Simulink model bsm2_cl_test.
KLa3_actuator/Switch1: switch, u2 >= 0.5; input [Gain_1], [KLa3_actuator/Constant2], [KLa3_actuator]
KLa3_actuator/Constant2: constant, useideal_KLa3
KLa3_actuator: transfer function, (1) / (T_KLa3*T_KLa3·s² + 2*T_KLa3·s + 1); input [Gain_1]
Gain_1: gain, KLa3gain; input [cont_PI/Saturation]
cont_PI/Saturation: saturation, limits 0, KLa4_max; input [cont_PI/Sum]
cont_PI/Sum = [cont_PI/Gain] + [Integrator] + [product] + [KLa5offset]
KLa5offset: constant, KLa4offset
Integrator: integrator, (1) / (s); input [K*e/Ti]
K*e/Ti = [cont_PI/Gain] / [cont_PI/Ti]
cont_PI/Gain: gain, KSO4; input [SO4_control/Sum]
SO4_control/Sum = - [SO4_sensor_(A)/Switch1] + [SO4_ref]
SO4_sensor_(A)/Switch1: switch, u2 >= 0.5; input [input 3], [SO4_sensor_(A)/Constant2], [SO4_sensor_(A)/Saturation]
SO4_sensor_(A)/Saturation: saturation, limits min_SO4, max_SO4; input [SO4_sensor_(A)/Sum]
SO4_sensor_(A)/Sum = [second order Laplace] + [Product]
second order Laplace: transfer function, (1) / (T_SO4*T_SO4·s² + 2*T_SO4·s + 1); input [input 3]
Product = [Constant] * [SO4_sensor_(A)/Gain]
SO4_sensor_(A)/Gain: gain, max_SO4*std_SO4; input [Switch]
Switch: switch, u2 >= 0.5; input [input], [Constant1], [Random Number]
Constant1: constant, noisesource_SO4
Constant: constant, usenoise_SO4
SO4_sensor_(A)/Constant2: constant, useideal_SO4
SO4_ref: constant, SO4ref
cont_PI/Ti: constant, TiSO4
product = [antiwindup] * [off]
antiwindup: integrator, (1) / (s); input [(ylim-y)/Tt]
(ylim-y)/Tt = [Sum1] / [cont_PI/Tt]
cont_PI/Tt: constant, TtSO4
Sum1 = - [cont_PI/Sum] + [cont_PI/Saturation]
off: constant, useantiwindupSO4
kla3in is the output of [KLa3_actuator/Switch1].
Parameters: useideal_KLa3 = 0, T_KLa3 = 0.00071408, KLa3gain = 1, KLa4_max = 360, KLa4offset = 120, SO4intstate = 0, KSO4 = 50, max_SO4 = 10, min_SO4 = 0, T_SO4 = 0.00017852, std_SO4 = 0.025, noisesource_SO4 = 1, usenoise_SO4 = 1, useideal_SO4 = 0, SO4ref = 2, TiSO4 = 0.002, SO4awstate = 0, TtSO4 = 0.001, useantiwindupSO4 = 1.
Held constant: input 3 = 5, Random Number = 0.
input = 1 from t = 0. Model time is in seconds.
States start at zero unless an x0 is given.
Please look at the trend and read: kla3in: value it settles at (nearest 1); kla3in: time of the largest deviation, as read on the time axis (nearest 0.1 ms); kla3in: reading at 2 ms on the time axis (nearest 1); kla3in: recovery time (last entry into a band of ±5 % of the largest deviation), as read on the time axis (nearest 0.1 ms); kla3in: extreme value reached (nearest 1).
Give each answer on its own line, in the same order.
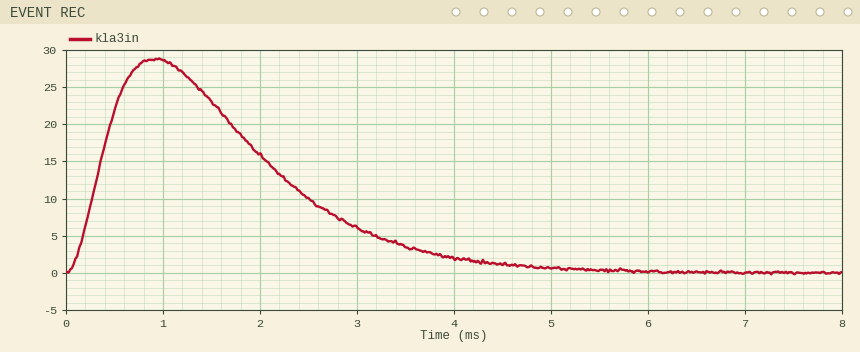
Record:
0
0.9 ms
16
4.3 ms
29
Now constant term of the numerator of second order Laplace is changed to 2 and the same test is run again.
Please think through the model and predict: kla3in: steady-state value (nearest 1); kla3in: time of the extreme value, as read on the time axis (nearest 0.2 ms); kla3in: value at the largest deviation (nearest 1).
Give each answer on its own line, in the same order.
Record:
0
0.8 ms
16
